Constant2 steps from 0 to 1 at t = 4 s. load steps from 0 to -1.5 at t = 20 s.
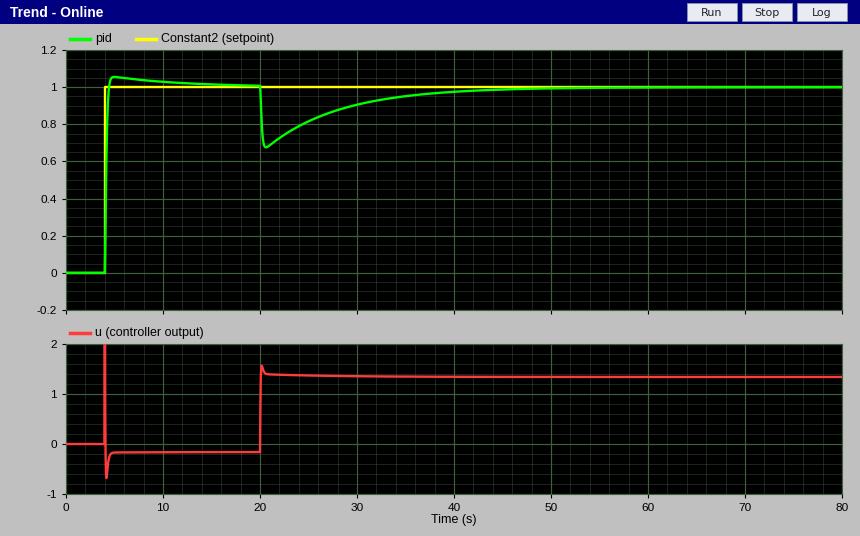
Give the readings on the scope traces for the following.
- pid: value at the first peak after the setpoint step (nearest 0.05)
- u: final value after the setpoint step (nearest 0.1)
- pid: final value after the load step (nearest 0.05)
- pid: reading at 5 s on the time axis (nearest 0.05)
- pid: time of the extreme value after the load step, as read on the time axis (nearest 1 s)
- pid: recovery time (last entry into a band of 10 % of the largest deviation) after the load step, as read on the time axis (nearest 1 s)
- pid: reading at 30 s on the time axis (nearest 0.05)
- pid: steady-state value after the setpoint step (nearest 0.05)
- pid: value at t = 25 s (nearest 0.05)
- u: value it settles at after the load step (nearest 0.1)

1.05
-0.2
1.00
1.05
21 s
38 s
0.90
1.00
0.80
1.3
